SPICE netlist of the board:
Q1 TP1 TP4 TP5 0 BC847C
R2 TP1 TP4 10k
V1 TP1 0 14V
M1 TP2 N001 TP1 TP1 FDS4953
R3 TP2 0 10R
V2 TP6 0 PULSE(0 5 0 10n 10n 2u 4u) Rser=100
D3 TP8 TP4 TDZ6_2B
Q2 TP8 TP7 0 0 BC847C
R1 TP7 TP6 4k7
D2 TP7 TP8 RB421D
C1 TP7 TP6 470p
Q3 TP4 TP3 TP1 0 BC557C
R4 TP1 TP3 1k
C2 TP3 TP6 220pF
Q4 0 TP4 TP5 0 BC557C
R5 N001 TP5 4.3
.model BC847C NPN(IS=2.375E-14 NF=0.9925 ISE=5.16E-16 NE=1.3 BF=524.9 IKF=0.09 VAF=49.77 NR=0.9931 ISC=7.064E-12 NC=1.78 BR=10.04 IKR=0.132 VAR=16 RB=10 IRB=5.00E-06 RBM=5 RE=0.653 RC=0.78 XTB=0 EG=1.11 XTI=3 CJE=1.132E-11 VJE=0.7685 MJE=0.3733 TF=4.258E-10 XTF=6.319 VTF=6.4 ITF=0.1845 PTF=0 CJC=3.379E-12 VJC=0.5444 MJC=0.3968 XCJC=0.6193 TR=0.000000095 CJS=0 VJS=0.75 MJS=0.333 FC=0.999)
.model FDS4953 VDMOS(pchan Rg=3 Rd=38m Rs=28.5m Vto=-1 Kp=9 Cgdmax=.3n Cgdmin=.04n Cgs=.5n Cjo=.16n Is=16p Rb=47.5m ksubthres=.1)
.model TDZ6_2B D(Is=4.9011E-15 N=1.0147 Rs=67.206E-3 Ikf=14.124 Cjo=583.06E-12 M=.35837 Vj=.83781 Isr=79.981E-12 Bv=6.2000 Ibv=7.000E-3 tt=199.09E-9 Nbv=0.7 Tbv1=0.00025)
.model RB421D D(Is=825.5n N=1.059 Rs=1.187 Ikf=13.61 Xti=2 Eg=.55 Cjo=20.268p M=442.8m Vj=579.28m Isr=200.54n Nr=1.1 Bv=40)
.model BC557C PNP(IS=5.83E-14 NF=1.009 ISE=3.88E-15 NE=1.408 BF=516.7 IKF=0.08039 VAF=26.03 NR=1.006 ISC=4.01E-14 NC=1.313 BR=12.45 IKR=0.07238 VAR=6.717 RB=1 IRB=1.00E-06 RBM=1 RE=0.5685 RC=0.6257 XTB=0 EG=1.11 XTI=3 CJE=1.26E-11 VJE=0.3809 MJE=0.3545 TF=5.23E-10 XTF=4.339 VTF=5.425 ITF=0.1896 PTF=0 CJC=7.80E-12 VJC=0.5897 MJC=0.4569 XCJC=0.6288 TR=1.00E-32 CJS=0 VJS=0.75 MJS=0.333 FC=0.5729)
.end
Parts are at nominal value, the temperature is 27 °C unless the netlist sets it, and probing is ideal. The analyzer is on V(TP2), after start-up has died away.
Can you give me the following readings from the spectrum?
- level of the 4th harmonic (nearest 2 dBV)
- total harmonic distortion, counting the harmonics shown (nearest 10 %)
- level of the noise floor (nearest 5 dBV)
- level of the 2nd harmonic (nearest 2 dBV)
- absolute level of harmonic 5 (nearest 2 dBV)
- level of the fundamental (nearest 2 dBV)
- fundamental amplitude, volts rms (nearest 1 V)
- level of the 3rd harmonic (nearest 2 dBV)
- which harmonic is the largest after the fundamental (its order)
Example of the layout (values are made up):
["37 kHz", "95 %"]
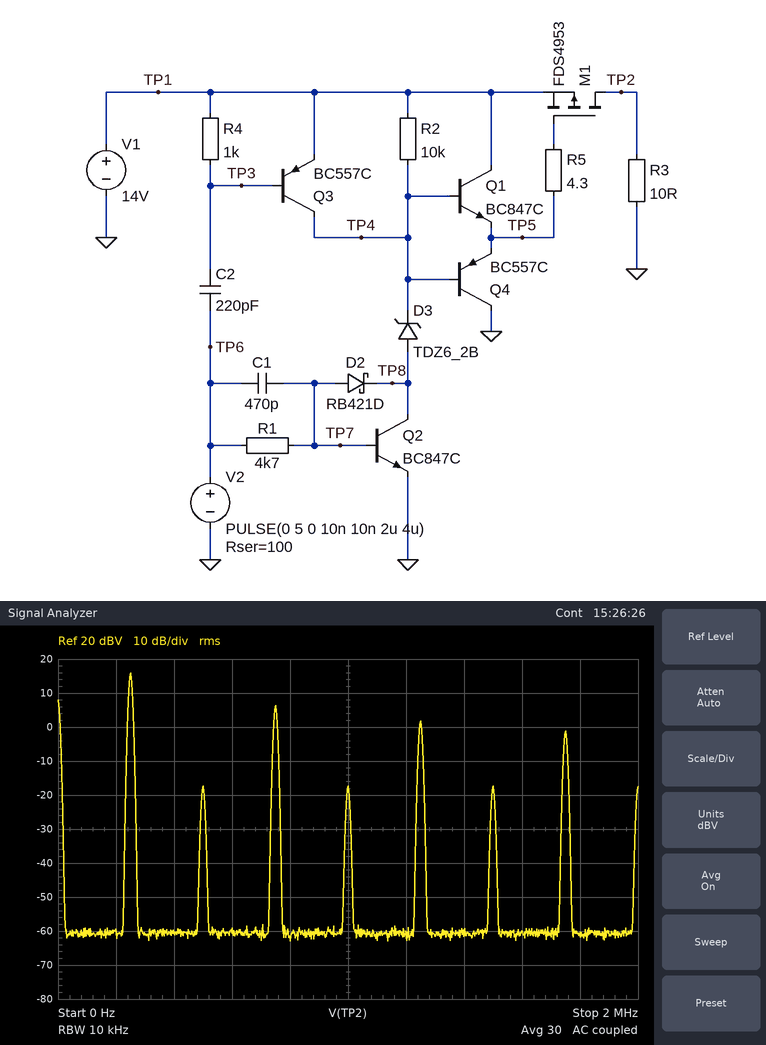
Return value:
["-18 dBV", "40 %", "-60 dBV", "-18 dBV", "2 dBV", "16 dBV", "6 V", "6 dBV", "3"]
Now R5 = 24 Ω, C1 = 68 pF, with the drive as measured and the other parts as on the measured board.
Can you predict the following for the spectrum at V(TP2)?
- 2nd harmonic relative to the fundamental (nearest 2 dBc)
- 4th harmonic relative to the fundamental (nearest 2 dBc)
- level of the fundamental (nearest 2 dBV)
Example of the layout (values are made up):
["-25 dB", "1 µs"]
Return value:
["-24 dBc", "-24 dBc", "16 dBV"]
